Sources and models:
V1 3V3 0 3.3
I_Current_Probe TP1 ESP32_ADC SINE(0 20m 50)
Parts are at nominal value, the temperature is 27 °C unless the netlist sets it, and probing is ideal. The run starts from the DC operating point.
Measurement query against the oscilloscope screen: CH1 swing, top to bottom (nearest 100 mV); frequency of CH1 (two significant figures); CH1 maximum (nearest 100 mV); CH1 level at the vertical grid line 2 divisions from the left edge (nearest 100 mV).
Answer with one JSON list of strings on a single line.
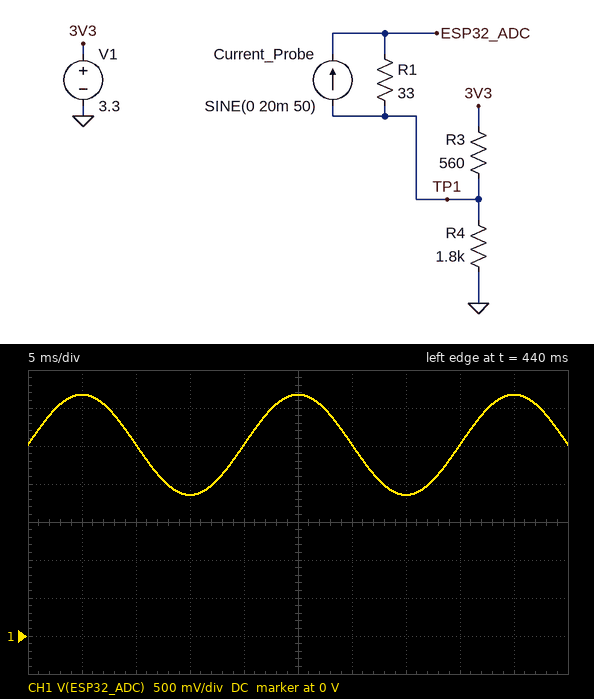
["1.3 V", "50 Hz", "3.2 V", "2.5 V"]
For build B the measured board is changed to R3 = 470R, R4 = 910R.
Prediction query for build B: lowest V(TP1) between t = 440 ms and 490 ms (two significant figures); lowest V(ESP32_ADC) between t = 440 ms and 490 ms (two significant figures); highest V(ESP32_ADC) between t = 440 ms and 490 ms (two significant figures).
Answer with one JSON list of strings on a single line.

["2.2 V", "1.5 V", "2.8 V"]
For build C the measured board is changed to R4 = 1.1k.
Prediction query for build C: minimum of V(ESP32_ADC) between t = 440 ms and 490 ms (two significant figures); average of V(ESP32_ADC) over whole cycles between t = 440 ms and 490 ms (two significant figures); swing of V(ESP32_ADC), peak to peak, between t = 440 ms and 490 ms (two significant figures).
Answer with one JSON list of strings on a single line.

["1.5 V", "2.2 V", "1.3 V"]
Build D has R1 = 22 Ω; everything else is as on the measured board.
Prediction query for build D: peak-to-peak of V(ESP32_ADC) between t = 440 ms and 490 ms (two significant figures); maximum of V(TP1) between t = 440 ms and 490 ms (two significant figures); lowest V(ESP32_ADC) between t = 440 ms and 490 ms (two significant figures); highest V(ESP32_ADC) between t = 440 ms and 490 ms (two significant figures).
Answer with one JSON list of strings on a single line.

["880 mV", "2.5 V", "2.1 V", "3.0 V"]
